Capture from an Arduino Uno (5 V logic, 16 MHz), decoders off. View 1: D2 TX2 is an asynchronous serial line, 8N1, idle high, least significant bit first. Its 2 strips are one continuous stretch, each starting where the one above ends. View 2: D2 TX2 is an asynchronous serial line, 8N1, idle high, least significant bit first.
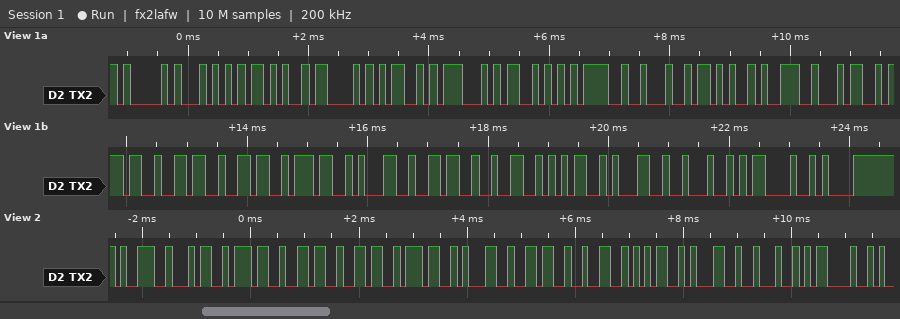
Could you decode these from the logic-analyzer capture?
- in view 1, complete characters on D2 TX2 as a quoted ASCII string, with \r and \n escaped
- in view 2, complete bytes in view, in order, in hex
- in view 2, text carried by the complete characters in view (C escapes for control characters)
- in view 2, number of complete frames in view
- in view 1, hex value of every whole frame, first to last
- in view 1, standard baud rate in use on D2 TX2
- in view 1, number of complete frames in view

"AT+CMGS=\"+94766716251\"\r\n"
39 34 37 36 36 37 31 36 32 35 31 22 0D
"94766716251\"\r"
13
41 54 2B 43 4D 47 53 3D 22 2B 39 34 37 36 36 37 31 36 32 35 31 22 0D 0A
9600 baud
24
